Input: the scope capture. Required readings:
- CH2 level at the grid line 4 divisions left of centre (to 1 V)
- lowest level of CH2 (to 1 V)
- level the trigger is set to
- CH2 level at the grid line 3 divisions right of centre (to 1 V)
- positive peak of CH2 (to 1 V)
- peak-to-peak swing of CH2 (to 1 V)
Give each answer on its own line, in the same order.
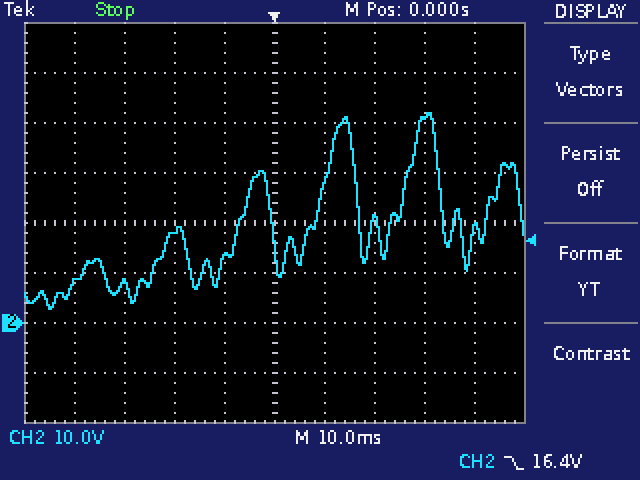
8 V
3 V
16.4 V
41 V
42 V
39 V
